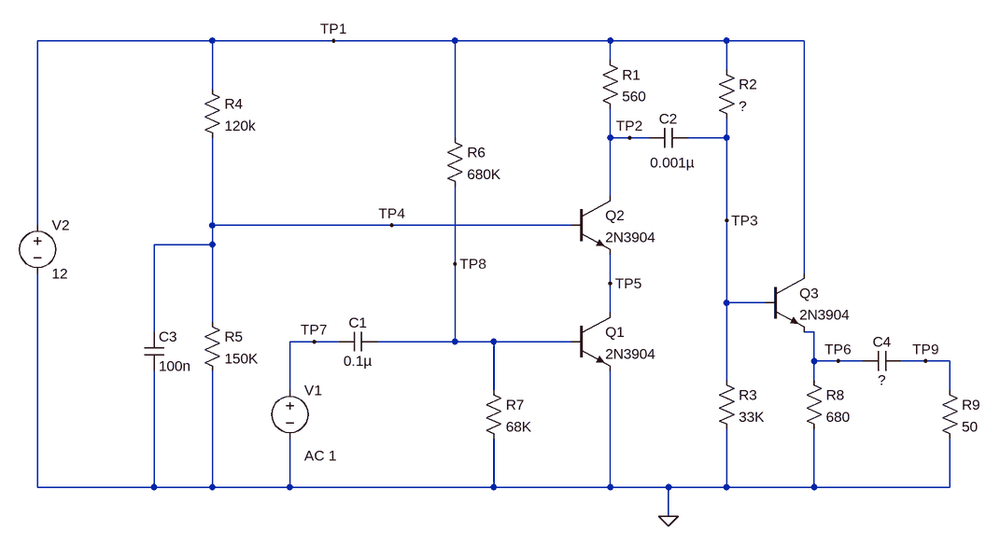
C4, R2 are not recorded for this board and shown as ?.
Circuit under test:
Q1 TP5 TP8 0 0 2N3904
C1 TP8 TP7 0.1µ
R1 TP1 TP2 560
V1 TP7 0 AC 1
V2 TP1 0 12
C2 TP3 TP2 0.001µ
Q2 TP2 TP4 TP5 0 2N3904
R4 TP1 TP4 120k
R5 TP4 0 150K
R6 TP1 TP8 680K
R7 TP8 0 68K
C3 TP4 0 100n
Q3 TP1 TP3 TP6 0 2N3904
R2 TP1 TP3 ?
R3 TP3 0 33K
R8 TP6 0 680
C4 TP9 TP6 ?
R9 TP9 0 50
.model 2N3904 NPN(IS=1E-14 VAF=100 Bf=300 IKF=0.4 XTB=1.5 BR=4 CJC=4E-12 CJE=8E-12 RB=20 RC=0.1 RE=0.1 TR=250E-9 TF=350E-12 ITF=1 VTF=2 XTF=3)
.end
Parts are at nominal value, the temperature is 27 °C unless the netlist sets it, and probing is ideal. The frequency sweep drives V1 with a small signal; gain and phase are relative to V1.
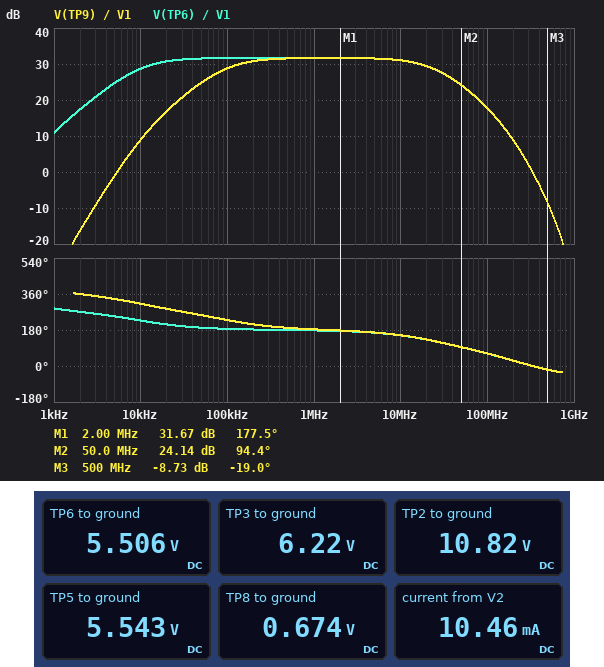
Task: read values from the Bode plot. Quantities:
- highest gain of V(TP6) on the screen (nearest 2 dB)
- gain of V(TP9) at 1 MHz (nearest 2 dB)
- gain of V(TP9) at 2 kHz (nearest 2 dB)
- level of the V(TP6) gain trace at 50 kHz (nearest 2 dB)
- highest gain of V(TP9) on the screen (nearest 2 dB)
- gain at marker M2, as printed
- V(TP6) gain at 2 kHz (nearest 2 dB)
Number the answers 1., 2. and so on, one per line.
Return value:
1. 32 dB
2. 32 dB
3. -16 dB
4. 32 dB
5. 32 dB
6. 24.14 dB
7. 18 dB
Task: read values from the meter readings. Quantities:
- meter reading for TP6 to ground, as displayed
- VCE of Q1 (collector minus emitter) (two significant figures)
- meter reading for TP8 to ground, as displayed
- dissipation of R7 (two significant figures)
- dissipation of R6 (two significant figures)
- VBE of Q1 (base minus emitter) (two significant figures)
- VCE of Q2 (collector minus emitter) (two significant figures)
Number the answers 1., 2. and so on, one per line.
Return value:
1. 5.506 V
2. 5.5 V
3. 0.674 V
4. 6.7 µW
5. 190 µW
6. 670 mV
7. 5.3 V
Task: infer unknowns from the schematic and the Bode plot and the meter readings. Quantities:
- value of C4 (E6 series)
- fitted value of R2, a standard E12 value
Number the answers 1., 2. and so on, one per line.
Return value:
1. 33 nF
2. 27 kΩ
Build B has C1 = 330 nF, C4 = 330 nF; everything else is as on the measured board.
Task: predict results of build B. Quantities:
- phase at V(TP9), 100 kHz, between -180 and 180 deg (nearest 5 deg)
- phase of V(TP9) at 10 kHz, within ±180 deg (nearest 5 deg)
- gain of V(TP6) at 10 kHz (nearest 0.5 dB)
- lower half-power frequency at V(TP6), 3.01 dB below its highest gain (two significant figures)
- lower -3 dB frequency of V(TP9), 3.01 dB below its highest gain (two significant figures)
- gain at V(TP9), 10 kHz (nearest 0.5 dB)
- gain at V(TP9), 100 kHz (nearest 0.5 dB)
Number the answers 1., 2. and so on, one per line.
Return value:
1. -165 deg
2. -90 deg
3. 25.5 dB
4. 21 kHz
5. 25 kHz
6. 22.5 dB
7. 31.5 dB
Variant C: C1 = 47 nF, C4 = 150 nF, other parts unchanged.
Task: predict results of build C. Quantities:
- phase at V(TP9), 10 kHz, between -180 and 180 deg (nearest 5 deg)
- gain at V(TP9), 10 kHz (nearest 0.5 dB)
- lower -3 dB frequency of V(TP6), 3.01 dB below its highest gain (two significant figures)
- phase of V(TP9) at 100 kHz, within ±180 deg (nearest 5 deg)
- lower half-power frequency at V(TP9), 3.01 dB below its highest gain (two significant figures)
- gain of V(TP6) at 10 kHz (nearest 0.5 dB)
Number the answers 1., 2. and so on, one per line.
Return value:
1. -70 deg
2. 19.5 dB
3. 18 kHz
4. -160 deg
5. 33 kHz
6. 27.0 dB
